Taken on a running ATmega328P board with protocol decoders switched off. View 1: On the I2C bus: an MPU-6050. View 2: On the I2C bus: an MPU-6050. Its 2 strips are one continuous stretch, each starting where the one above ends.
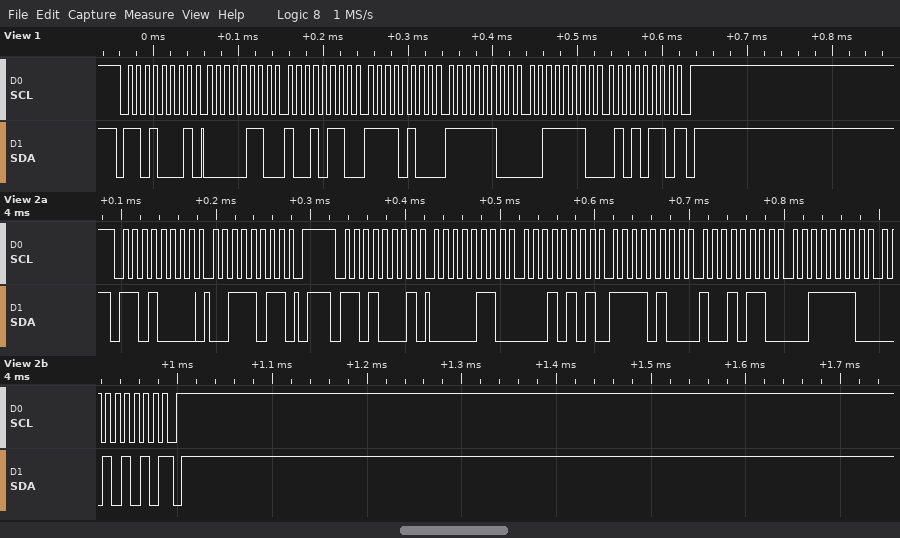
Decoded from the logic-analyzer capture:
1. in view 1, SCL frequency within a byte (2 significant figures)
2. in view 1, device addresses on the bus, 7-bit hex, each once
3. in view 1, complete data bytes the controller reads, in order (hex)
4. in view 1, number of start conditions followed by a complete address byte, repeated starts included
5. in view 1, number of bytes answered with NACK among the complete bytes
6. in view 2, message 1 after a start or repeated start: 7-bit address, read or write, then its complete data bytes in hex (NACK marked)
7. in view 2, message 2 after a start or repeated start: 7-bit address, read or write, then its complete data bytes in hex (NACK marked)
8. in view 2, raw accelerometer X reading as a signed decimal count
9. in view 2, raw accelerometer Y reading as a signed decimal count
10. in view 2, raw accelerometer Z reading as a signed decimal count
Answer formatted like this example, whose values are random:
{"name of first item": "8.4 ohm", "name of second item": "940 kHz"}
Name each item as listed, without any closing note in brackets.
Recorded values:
{"in view 1, SCL frequency within a byte": "100 kHz", "in view 1, device addresses on the bus, 7-bit hex, each once": "0x68", "in view 1, complete data bytes the controller reads, in order": "06 96 F4 FC 3E 56", "in view 1, number of start conditions followed by a complete address byte, repeated starts included": "1", "in view 1, number of bytes answered with NACK among the complete bytes": "1", "in view 2, message 1 after a start or repeated start: 7-bit address, read or write, then its complete data bytes in hex": "0x68 write: 3B", "in view 2, message 2 after a start or repeated start: 7-bit address, read or write, then its complete data bytes in hex": "0x68 read: 06 15 F4 96 3E 2A NACK", "in view 2, raw accelerometer X reading as a signed decimal count": "1557", "in view 2, raw accelerometer Y reading as a signed decimal count": "-2922", "in view 2, raw accelerometer Z reading as a signed decimal count": "15914"}
